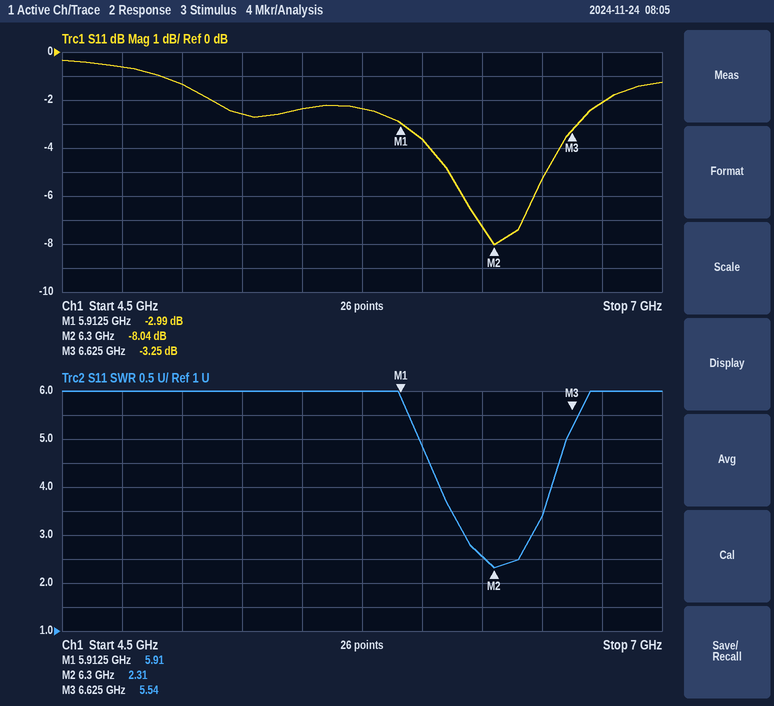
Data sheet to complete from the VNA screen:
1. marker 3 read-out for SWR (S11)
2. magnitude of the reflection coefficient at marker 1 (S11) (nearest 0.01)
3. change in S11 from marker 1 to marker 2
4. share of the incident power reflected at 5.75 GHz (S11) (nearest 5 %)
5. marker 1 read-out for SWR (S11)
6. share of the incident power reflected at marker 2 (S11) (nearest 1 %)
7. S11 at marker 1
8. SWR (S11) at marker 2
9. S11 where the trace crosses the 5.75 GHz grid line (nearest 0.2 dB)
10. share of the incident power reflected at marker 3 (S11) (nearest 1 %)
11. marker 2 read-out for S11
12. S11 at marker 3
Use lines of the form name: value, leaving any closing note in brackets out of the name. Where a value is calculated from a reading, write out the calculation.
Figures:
marker 3 read-out for SWR: 5.54
magnitude of the reflection coefficient at marker 1 (S11): 10^(-2.99/20) ≈ 0.71
change in S11 from marker 1 to marker 2: -8.04 − (-2.99) = -5.05 dB
share of the incident power reflected at 5.75 GHz (S11): 10^(-2.4/10) ≈ 57.5 %, so 60 % to the nearest 5 %
marker 1 read-out for SWR: 5.91
share of the incident power reflected at marker 2 (S11): 10^(-8.04/10) ≈ 16 %
S11 at marker 1: -2.99 dB
SWR (S11) at marker 2: 2.31
S11 where the trace crosses the 5.75 GHz grid line: -2.4 dB
share of the incident power reflected at marker 3 (S11): 10^(-3.25/10) ≈ 47 %
marker 2 read-out for S11: -8.04 dB
S11 at marker 3: -3.25 dB
